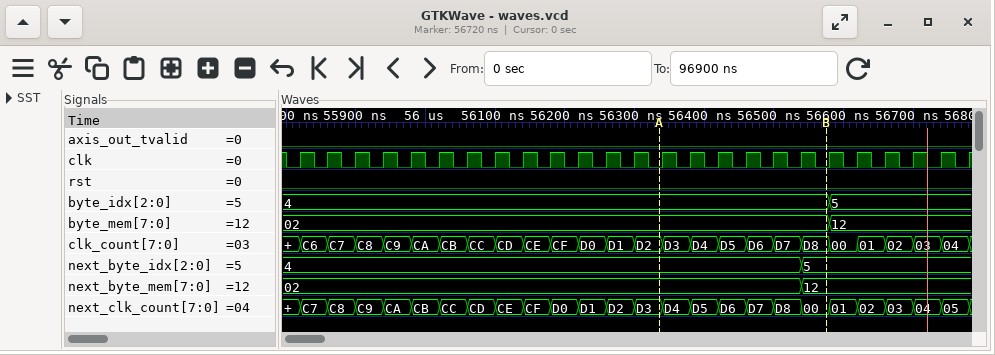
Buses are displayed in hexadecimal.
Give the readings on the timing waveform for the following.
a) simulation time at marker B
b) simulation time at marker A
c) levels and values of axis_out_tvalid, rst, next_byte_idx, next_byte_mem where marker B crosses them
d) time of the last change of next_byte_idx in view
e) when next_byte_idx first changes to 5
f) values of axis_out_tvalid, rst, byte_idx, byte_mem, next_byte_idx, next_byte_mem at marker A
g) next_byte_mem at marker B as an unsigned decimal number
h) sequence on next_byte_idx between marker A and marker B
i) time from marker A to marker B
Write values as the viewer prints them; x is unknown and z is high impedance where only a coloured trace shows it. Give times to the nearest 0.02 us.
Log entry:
56.58 us
56.34 us
axis_out_tvalid=0, rst=0, next_byte_idx=5, next_byte_mem=12
56.54 us
56.54 us
axis_out_tvalid=0, rst=0, byte_idx=4, byte_mem=02, next_byte_idx=4, next_byte_mem=02
18
4, 5
0.24 us
